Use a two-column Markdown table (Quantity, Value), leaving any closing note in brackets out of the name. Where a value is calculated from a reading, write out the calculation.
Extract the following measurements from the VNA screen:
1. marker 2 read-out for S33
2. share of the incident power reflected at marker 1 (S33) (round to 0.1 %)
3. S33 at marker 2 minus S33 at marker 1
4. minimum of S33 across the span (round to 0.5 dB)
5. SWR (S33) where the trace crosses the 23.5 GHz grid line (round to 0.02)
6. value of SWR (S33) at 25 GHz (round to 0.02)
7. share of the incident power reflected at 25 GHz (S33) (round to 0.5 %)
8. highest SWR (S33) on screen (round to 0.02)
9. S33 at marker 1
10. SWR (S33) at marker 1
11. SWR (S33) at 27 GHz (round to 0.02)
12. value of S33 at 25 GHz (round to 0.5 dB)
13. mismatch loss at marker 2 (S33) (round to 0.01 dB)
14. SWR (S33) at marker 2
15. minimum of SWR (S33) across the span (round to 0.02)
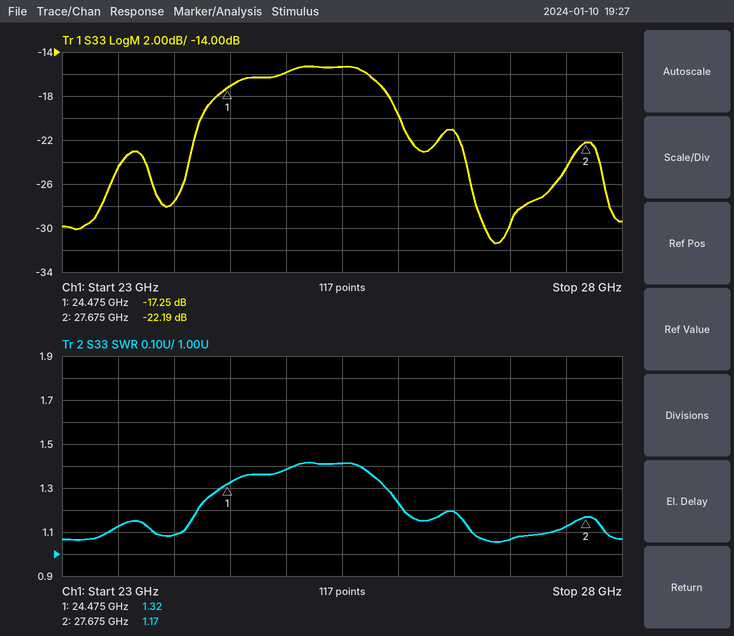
| Quantity | Value |
|---|---|
| marker 2 read-out for S33 | -22.19 dB |
| share of the incident power reflected at marker 1 (S33) | 10^(-17.25/10) ≈ 1.9 % |
| S33 at marker 2 minus S33 at marker 1 | -22.19 − (-17.25) = -4.94 dB |
| minimum of S33 across the span | -31.5 dB |
| SWR (S33) where the trace crosses the 23.5 GHz grid line | 1.12 |
| value of SWR (S33) at 25 GHz | 1.38 |
| share of the incident power reflected at 25 GHz (S33) | 10^(-16/10) ≈ 2.5 % |
| highest SWR (S33) on screen | 1.42 |
| S33 at marker 1 | -17.25 dB |
| SWR (S33) at marker 1 | 1.32 |
| SWR (S33) at 27 GHz | 1.06 |
| value of S33 at 25 GHz | -16.0 dB |
| mismatch loss at marker 2 (S33) | −10 log10(1 − 10^(-22.19/10)) ≈ 0.03 dB |
| SWR (S33) at marker 2 | 1.17 |
| minimum of SWR (S33) across the span | 1.06 |
